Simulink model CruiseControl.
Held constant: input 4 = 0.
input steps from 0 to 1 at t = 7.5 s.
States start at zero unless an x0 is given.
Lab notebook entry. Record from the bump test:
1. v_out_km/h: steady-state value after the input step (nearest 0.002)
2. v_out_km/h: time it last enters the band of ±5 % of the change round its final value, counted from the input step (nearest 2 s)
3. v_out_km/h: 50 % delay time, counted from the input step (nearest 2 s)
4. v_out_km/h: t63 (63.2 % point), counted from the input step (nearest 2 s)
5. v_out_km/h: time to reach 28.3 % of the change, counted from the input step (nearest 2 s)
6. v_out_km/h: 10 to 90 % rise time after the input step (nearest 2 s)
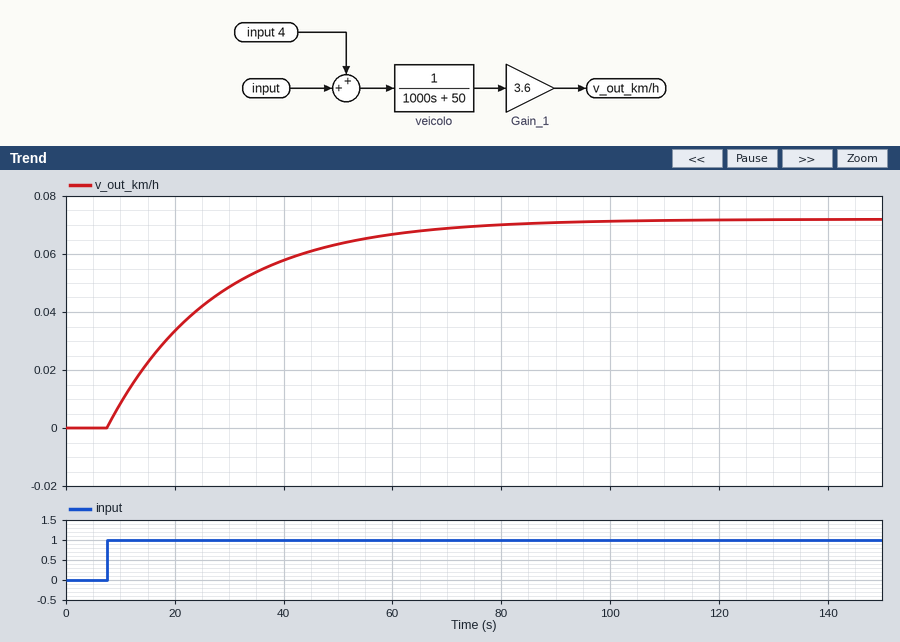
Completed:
0.072
60 s
14 s
20 s
6 s
44 s
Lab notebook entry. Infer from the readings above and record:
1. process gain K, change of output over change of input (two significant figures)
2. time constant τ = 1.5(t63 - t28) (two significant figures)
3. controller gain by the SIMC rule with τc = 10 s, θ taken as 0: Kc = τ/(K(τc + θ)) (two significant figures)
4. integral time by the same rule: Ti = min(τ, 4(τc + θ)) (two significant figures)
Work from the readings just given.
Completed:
0.072
21 s
29
21 s
